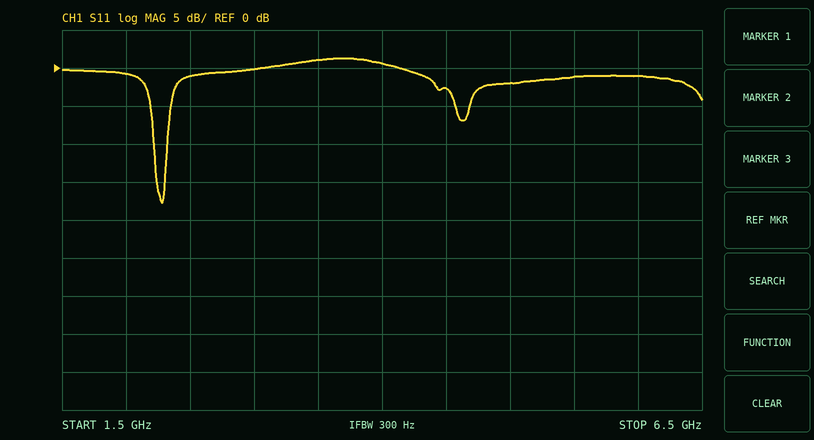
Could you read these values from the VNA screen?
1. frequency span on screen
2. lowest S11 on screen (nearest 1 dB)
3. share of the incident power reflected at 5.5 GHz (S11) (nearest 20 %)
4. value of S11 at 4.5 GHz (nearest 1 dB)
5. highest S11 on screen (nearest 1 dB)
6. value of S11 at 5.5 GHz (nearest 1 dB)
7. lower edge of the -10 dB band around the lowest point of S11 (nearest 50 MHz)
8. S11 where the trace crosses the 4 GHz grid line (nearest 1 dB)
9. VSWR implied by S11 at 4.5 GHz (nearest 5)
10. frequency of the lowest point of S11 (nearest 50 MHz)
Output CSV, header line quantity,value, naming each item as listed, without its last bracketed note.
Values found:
quantity,value
frequency span on screen,5 GHz
lowest S11 on screen,-18 dB
share of the incident power reflected at 5.5 GHz (S11),80 %
value of S11 at 4.5 GHz,-3 dB
highest S11 on screen,1 dB
value of S11 at 5.5 GHz,-1 dB
lower edge of the -10 dB band around the lowest point of S11,2.20 GHz
S11 where the trace crosses the 4 GHz grid line,1 dB
VSWR implied by S11 at 4.5 GHz,5
frequency of the lowest point of S11,2.30 GHz
